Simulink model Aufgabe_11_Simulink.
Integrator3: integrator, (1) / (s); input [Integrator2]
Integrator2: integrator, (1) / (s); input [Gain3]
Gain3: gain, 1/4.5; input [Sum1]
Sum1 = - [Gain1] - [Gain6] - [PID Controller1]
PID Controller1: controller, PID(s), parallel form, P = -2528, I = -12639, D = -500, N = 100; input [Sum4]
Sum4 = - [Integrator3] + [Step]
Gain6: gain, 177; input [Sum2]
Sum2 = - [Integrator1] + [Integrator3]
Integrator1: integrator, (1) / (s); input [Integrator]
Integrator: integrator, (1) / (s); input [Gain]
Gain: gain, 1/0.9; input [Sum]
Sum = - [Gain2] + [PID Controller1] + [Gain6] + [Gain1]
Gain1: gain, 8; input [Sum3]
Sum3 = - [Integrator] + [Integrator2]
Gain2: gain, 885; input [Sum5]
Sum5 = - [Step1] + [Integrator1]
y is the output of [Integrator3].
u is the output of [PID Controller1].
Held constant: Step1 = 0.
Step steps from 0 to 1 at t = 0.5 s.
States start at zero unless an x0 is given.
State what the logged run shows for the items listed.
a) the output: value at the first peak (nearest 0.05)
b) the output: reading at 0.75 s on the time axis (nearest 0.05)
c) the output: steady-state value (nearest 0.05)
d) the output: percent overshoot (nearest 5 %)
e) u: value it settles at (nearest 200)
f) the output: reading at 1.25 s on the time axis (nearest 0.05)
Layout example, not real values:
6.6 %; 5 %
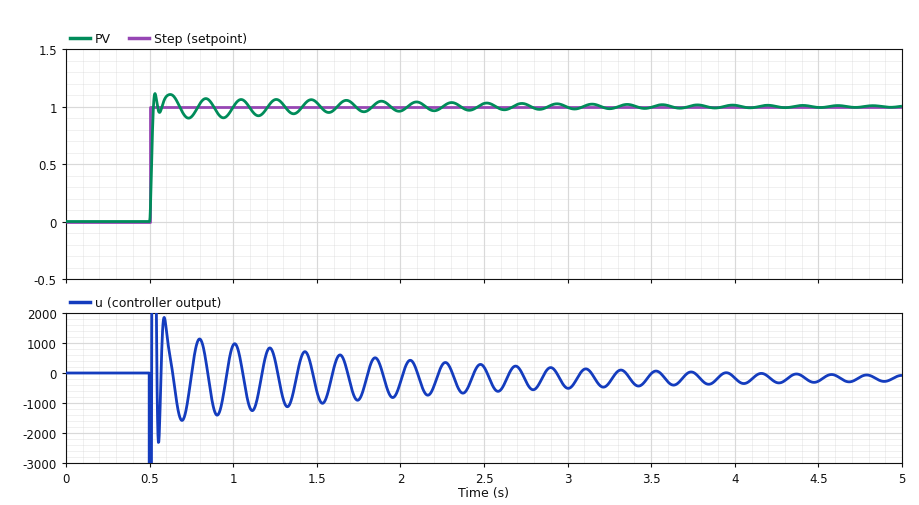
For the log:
1.10; 0.90; 1.00; 10 %; -200; 1.05
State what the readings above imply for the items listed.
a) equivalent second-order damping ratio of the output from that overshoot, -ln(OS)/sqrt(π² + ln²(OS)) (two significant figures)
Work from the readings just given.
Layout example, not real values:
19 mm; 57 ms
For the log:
0.59
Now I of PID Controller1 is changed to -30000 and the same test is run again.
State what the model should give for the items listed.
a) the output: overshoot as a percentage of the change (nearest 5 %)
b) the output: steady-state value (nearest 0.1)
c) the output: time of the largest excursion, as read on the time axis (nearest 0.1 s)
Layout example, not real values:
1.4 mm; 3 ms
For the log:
15 %; 1.0; 0.6 s
